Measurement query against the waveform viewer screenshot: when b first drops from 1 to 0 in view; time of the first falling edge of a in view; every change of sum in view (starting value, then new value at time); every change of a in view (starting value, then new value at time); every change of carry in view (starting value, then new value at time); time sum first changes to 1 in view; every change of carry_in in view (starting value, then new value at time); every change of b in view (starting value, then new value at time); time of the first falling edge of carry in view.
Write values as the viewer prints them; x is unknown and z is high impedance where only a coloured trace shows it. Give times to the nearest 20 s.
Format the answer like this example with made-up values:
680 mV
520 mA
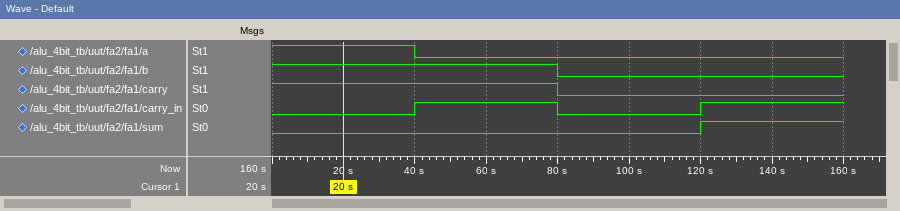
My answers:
80 s
40 s
0, 1 at 120 s
1, 0 at 40 s
1, 0 at 80 s
120 s
0, 1 at 40 s, 0 at 80 s, 1 at 120 s
1, 0 at 80 s
80 s
